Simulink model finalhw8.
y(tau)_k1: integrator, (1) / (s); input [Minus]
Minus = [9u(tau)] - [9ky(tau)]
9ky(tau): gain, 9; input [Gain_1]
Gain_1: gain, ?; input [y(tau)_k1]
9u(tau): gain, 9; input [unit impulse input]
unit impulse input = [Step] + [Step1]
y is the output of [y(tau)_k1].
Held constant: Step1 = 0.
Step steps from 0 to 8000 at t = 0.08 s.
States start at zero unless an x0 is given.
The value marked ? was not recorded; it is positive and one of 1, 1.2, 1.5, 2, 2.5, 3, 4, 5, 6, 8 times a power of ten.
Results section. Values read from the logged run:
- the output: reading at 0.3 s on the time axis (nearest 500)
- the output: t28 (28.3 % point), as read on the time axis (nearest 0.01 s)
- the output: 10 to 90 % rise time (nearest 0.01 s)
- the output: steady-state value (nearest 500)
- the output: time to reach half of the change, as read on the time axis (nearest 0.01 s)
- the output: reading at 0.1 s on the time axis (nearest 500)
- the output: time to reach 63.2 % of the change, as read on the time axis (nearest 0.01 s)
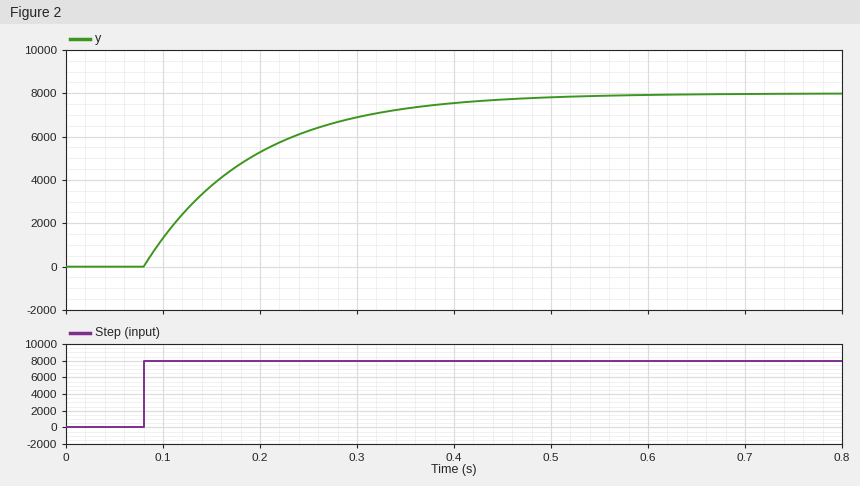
7000
0.12 s
0.24 s
8000
0.16 s
1500
0.19 s
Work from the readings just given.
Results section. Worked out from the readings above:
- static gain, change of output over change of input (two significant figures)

1.0
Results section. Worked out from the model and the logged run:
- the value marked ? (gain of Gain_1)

1
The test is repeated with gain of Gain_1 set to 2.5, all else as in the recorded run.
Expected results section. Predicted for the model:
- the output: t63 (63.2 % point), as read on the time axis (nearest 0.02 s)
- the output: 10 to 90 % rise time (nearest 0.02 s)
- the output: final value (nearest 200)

0.12 s
0.10 s
3200
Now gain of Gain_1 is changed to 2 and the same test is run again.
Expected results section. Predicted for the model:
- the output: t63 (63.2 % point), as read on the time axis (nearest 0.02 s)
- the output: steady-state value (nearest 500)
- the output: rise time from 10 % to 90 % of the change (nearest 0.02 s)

0.14 s
4000
0.12 s
